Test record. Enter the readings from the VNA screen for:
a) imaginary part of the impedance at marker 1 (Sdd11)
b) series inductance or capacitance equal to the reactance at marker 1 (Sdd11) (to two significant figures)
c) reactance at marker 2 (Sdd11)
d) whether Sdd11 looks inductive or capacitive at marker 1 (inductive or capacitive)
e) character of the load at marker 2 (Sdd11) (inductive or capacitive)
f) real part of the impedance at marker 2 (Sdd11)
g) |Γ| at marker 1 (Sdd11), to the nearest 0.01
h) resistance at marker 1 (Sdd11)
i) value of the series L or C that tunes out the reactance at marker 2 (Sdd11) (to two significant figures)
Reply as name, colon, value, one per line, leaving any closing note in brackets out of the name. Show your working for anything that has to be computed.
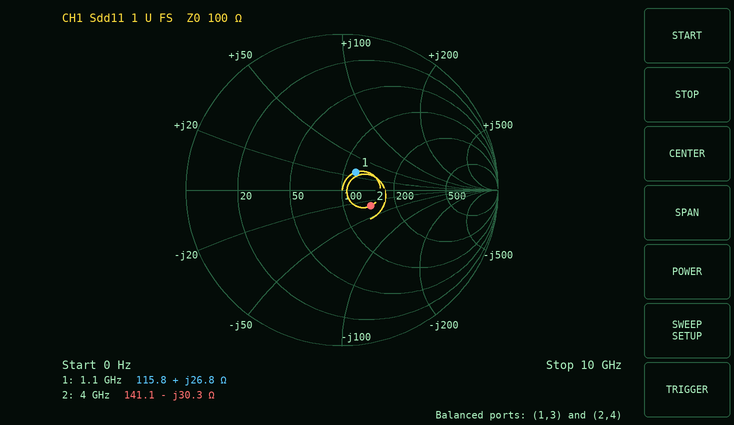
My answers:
imaginary part of the impedance at marker 1: +26.8 Ω
series inductance or capacitance equal to the reactance at marker 1 (Sdd11): L = 26.8 Ω/(2π × 1.1 GHz) ≈ 3.9 nH
reactance at marker 2: -30.3 Ω
whether Sdd11 looks inductive or capacitive at marker 1: inductive
character of the load at marker 2 (Sdd11): capacitive
real part of the impedance at marker 2: 141.1 Ω
|Γ| at marker 1 (Sdd11), to the nearest 0.01: 0.14
resistance at marker 1: 115.8 Ω
value of the series L or C that tunes out the reactance at marker 2 (Sdd11): L = 30.3 Ω/(2π × 4 GHz) ≈ 1.2 nH
